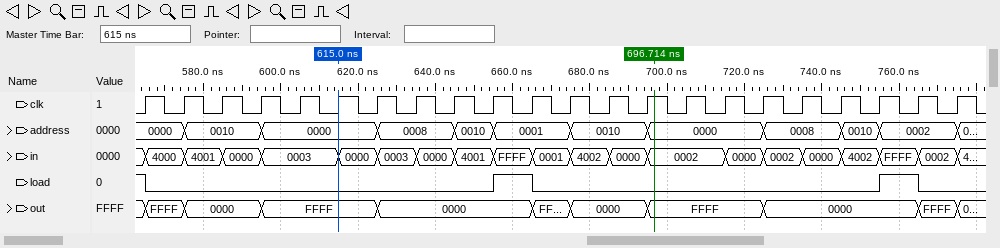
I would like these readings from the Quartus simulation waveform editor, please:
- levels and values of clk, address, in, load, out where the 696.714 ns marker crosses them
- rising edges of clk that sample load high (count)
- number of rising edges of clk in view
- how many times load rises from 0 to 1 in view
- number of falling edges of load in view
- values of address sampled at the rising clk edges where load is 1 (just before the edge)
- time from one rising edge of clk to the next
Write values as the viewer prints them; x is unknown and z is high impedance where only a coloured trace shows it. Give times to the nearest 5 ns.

clk=1, address=0000, in=0002, load=0, out=FFFF
3
22
2
3
0000, 0001, 0002
10 ns
